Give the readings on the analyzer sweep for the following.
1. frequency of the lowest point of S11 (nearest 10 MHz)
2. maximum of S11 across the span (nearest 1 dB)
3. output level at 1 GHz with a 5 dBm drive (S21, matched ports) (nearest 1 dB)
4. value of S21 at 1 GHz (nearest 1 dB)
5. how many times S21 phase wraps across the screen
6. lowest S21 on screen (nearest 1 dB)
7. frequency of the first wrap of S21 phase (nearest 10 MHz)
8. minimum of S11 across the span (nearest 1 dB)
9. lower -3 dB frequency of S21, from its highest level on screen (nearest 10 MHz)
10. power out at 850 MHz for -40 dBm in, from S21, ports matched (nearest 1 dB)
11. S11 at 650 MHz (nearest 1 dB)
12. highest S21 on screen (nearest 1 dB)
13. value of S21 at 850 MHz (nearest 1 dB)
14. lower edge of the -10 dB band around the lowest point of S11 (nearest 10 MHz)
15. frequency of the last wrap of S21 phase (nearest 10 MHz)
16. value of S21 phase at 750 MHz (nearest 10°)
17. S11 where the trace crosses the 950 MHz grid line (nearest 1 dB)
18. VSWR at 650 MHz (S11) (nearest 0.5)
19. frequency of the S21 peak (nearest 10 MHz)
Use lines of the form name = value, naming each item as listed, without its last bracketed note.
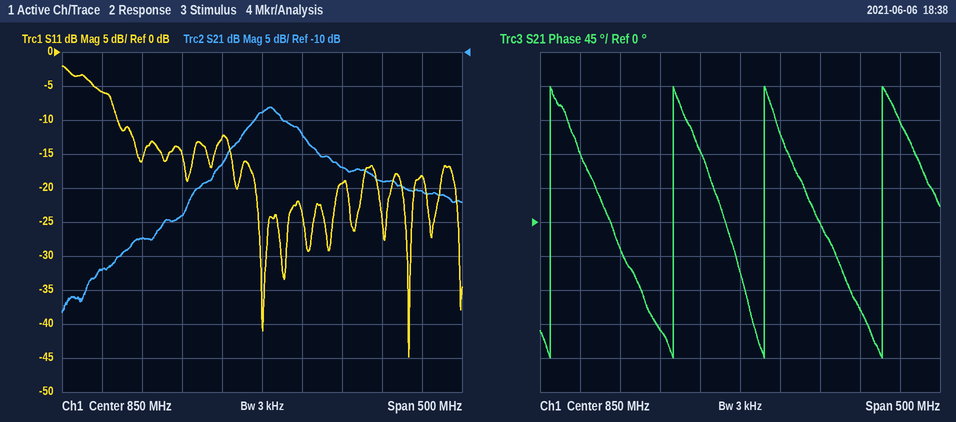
frequency of the lowest point of S11 = 1.03 GHz
maximum of S11 across the span = -2 dB
output level at 1 GHz with a 5 dBm drive (S21, matched ports) = -24 dBm
value of S21 at 1 GHz = -29 dB
how many times S21 phase wraps across the screen = 4
lowest S21 on screen = -48 dB
frequency of the first wrap of S21 phase = 610 MHz
minimum of S11 across the span = -45 dB
lower -3 dB frequency of S21, from its highest level on screen = 830 MHz
power out at 850 MHz for -40 dBm in, from S21, ports matched = -59 dBm
S11 at 650 MHz = -6 dB
highest S21 on screen = -18 dB
value of S21 at 850 MHz = -19 dB
lower edge of the -10 dB band around the lowest point of S11 = 670 MHz
frequency of the last wrap of S21 phase = 1.03 GHz
value of S21 phase at 750 MHz = -140°
S11 where the trace crosses the 950 MHz grid line = -19 dB
VSWR at 650 MHz (S11) = 3.0
frequency of the S21 peak = 860 MHz
